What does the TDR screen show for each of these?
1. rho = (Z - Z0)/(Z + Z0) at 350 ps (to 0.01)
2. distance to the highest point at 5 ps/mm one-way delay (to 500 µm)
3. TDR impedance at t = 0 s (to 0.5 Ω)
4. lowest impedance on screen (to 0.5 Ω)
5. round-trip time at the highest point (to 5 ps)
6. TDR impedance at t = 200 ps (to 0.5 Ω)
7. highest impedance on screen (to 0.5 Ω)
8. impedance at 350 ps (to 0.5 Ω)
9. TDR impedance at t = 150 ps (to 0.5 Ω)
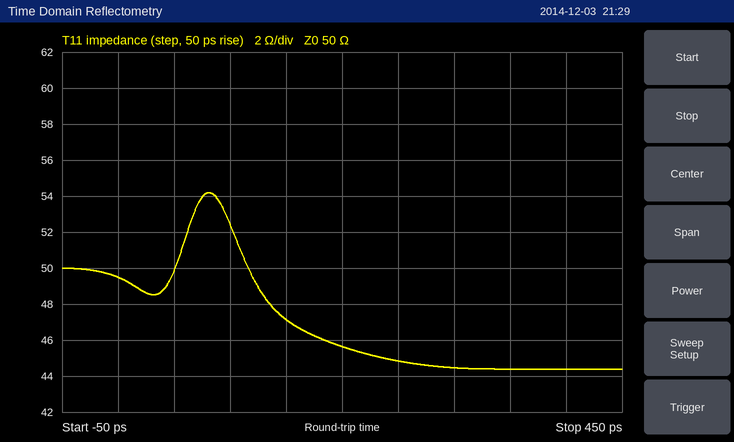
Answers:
-0.06
8.0 mm
49.5 Ω
44.5 Ω
80 ps
45.5 Ω
54.0 Ω
44.5 Ω
47.0 Ω
